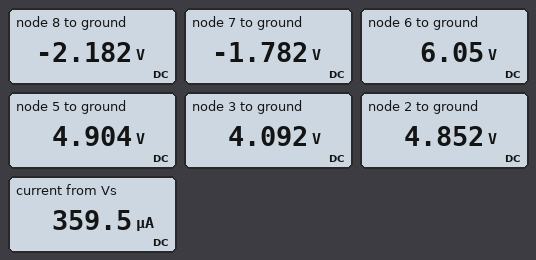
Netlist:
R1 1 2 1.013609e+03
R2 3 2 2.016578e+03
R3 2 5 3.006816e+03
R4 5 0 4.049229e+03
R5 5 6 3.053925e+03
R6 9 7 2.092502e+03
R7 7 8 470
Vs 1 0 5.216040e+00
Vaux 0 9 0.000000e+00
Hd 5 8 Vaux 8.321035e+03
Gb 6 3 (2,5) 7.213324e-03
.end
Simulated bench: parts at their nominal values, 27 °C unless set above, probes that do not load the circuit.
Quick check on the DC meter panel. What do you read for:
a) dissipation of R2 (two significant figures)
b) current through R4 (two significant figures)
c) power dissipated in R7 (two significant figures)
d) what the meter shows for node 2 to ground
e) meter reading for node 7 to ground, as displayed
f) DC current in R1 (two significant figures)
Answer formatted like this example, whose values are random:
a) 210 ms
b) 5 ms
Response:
a) 290 µW
b) 1.2 mA
c) 340 µW
d) 4.852 V
e) -1.782 V
f) 360 µA
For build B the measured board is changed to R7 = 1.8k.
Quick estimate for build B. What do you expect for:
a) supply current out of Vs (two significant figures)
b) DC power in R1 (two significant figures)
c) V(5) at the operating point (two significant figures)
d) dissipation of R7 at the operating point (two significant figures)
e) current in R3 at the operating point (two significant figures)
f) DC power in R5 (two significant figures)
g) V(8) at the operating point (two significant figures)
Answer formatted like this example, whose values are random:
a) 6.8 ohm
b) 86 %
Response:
a) 110 µA
b) 12 µW
c) 5.1 V
d) 2.4 mW
e) 5.2 µA
f) 39 µW
g) -4.5 V
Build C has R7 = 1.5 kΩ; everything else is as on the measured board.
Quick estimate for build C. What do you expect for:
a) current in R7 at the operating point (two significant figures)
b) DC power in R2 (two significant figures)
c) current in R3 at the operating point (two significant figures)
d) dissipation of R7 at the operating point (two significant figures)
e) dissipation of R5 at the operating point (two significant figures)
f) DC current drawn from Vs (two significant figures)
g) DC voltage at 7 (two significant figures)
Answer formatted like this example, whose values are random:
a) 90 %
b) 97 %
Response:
a) 1.1 mA
b) 71 µW
c) 8.7 µA
d) 1.7 mW
e) 110 µW
f) 180 µA
g) -2.2 V
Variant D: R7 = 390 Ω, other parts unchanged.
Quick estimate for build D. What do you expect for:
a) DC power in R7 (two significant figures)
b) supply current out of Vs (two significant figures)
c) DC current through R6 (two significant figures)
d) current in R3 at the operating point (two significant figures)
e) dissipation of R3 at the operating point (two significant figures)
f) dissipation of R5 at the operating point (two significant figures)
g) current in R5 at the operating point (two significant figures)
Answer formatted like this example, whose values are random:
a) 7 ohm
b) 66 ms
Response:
a) 270 µW
b) 370 µA
c) 840 µA
d) 18 µA
e) 960 nW
f) 460 µW
g) 390 µA
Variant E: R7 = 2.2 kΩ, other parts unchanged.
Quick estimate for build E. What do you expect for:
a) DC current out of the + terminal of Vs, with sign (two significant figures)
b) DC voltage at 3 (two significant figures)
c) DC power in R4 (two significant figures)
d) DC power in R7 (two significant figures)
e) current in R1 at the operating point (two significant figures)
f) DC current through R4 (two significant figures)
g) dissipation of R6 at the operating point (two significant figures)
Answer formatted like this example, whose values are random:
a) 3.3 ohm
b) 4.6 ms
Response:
a) -6.6 µA
b) 5.2 V
c) 6.7 mW
d) 3.7 mW
e) 6.6 µA
f) 1.3 mA
g) 3.5 mW
